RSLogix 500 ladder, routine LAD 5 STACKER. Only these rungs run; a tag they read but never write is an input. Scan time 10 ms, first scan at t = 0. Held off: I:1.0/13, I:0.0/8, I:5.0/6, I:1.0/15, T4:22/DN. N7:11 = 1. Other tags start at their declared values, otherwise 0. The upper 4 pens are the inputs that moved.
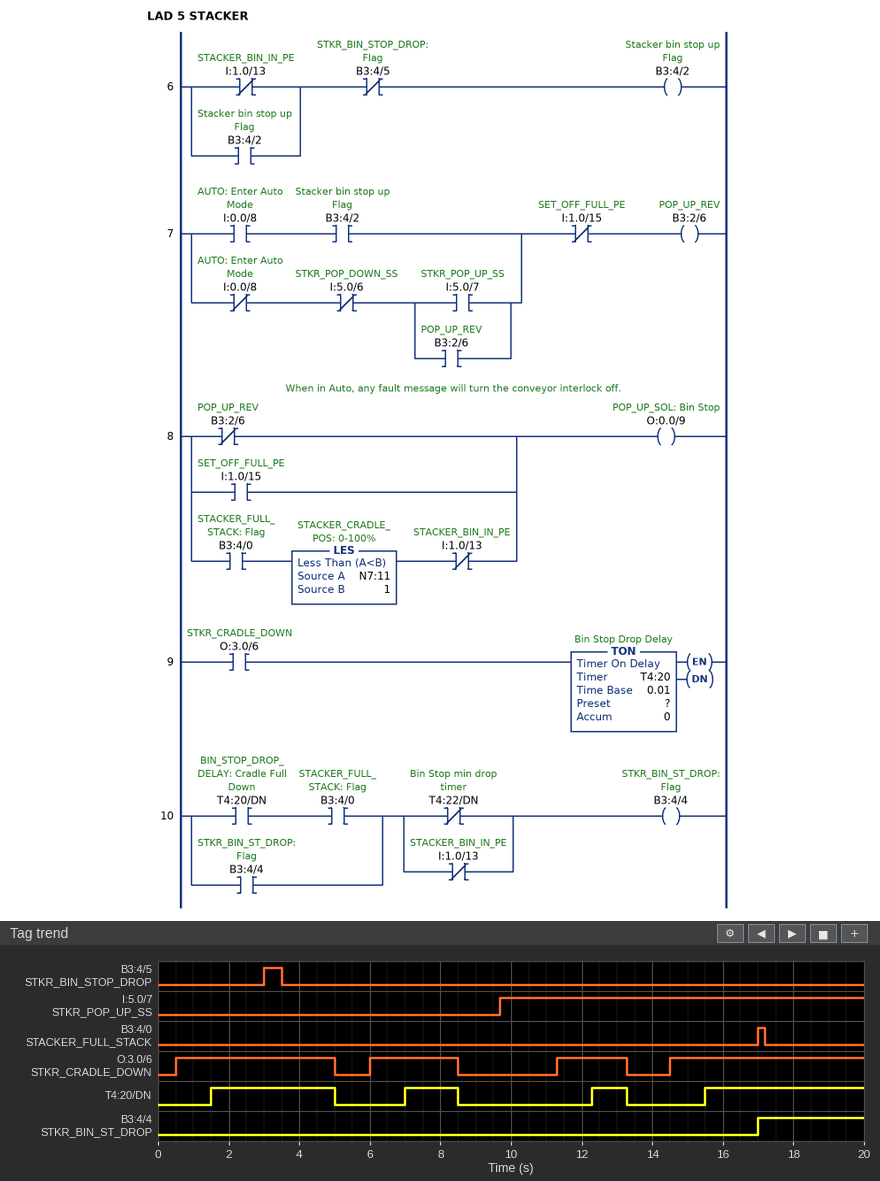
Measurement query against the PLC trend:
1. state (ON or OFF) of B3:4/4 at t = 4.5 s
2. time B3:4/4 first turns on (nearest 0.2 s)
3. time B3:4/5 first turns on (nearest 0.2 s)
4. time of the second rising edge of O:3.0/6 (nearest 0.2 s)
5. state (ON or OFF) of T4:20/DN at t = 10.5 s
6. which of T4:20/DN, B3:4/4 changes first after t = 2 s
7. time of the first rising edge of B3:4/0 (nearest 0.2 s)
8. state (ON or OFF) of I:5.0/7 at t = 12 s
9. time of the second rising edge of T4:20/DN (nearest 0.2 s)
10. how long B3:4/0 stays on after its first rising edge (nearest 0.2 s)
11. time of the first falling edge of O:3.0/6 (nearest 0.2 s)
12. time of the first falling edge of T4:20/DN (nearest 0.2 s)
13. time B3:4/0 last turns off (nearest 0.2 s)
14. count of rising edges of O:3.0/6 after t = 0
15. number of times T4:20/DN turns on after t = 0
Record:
OFF
17.0 s
3.0 s
6.0 s
OFF
T4:20/DN
17.0 s
ON
7.0 s
0.2 s
5.0 s
5.0 s
17.2 s
4
4
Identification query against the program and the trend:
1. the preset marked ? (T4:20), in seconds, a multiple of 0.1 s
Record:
1.0 s
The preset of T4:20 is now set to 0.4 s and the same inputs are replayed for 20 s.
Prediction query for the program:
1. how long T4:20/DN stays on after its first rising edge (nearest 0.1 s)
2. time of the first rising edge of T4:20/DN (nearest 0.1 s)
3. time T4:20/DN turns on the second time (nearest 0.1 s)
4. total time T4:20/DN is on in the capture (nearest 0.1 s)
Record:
4.1 s
0.9 s
6.4 s
12.9 s
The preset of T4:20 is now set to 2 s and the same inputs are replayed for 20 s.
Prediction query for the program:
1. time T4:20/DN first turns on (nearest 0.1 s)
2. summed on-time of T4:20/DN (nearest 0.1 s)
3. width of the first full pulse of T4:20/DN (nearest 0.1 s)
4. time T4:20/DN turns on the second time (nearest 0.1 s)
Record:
2.5 s
6.5 s
2.5 s
8.0 s
